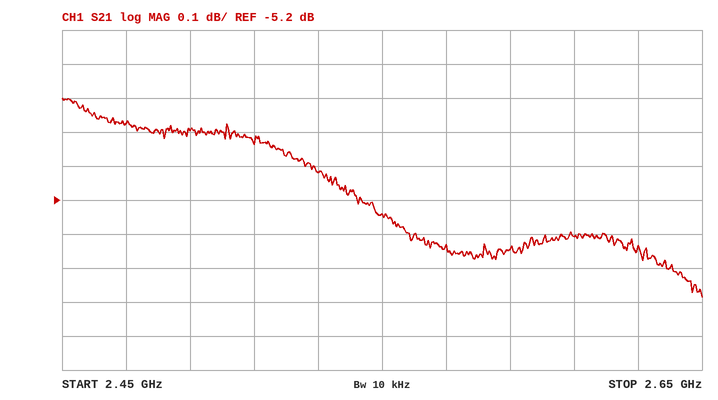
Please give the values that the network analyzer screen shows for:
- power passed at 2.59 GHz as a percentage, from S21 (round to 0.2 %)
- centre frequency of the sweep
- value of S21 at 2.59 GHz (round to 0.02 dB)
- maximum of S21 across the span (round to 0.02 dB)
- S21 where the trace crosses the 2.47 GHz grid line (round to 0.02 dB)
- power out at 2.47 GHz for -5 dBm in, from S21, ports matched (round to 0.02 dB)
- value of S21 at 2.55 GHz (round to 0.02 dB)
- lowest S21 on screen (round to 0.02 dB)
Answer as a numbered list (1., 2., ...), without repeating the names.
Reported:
1. 29.2 %
2. 2.55 GHz
3. -5.34 dB
4. -4.90 dB
5. -4.98 dB
6. -9.98 dBm
7. -5.24 dB
8. -5.48 dB
